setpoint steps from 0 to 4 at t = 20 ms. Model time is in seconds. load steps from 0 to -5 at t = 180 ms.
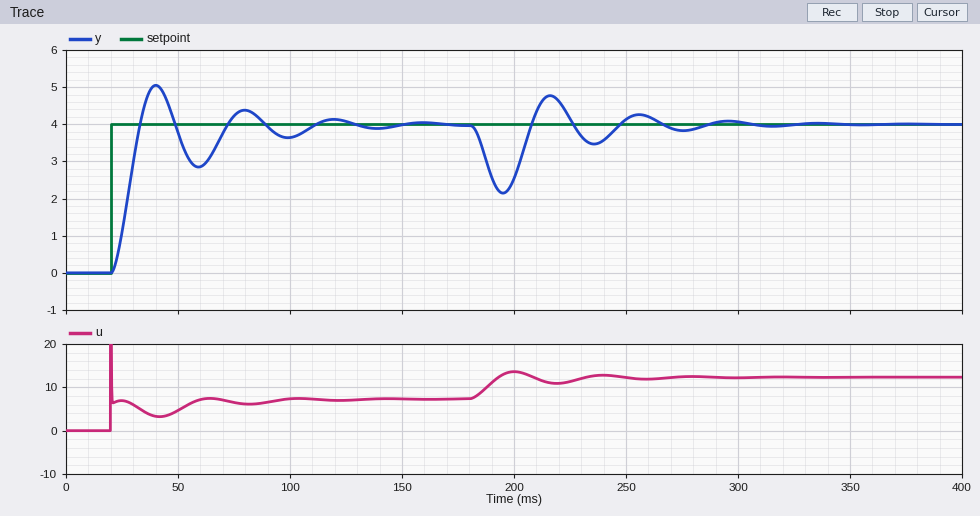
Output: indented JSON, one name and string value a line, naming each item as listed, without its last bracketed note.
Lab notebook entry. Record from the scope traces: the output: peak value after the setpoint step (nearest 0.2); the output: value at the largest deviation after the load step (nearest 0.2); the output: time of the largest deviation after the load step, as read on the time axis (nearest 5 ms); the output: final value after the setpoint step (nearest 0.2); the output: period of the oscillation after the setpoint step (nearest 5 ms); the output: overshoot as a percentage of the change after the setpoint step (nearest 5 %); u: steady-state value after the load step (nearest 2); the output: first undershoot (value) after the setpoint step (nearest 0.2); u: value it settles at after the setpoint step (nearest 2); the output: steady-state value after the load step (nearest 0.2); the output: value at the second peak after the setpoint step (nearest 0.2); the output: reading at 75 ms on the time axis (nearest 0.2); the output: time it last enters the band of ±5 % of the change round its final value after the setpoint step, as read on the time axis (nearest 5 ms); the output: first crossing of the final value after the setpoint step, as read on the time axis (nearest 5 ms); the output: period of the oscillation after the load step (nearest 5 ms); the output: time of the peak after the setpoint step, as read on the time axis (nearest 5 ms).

{
  "the output: peak value after the setpoint step": "5.0",
  "the output: value at the largest deviation after the load step": "2.2",
  "the output: time of the largest deviation after the load step, as read on the time axis": "195 ms",
  "the output: final value after the setpoint step": "4.0",
  "the output: period of the oscillation after the setpoint step": "40 ms",
  "the output: overshoot as a percentage of the change after the setpoint step": "25 %",
  "u: steady-state value after the load step": "12",
  "the output: first undershoot (value) after the setpoint step": "2.8",
  "u: value it settles at after the setpoint step": "8",
  "the output: steady-state value after the load step": "4.0",
  "the output: value at the second peak after the setpoint step": "4.4",
  "the output: reading at 75 ms on the time axis": "4.2",
  "the output: time it last enters the band of ±5 % of the change round its final value after the setpoint step, as read on the time axis": "105 ms",
  "the output: first crossing of the final value after the setpoint step, as read on the time axis": "35 ms",
  "the output: period of the oscillation after the load step": "40 ms",
  "the output: time of the peak after the setpoint step, as read on the time axis": "40 ms"
}
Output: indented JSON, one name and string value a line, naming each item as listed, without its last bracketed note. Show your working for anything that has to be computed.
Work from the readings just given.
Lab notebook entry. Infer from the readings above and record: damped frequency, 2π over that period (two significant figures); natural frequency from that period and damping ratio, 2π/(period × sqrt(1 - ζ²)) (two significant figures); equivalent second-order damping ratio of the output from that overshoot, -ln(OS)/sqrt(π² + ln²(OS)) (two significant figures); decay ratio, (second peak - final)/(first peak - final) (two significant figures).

{
  "damped frequency, 2π over that period": "2π / 40 = 0.16 rad/ms",
  "natural frequency from that period and damping ratio, 2π/(period × sqrt(1 - ζ²))": "2π / (40 × sqrt(1 - 0.4²)) = 0.17 rad/ms",
  "equivalent second-order damping ratio of the output from that overshoot, -ln(OS)/sqrt(π² + ln²(OS))": "ln(0.25) = -1.386; 1.386 / sqrt(9.870 + 1.922) = 0.40",
  "decay ratio, (second peak - final)/(first peak - final)": "(4.4 - 4) / (5 - 4) = 0.40"
}
